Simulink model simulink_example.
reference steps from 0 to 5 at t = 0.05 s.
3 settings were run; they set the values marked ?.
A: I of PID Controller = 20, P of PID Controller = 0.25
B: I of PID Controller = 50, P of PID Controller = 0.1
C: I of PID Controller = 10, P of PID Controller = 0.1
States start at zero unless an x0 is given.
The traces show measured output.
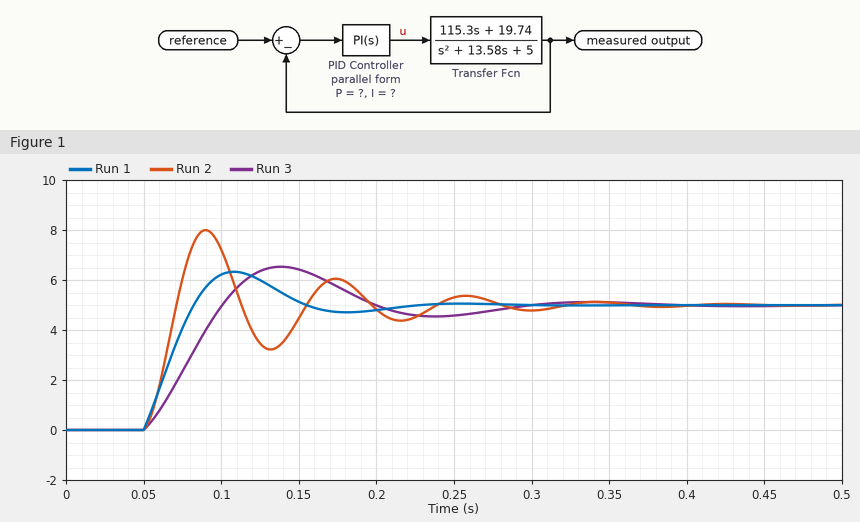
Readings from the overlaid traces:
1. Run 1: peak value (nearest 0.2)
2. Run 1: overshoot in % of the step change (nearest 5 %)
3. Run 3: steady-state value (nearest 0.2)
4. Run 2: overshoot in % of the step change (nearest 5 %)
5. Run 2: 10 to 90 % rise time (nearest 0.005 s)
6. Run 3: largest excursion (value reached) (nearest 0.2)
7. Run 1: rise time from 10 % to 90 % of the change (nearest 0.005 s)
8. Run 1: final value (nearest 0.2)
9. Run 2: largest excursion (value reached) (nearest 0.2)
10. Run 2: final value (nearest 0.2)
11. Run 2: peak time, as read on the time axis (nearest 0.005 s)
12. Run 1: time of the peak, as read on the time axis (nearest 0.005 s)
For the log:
6.4
25 %
5.0
60 %
0.015 s
6.6
0.025 s
5.0
8.0
5.0
0.090 s
0.110 s
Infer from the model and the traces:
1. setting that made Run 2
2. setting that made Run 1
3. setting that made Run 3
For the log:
B
A
C
